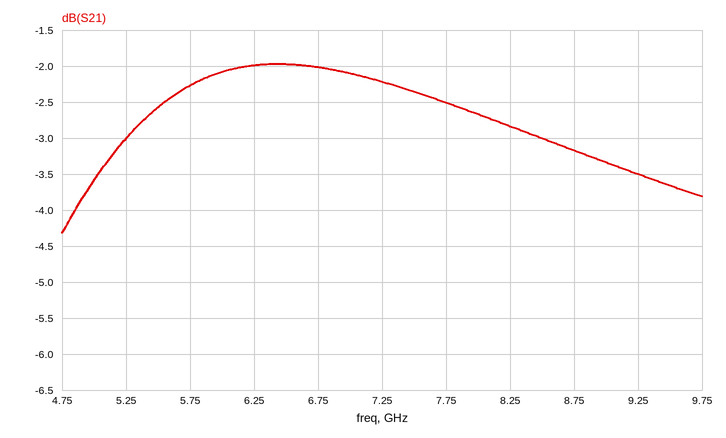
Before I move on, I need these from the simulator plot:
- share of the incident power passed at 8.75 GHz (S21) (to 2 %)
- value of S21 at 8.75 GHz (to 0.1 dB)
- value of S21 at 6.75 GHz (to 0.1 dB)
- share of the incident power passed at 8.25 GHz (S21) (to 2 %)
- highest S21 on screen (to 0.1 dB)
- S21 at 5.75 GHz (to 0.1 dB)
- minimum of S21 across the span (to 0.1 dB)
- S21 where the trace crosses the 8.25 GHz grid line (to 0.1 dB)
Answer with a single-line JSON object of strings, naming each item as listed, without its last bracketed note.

{"share of the incident power passed at 8.75 GHz (S21)": "48 %", "value of S21 at 8.75 GHz": "-3.2 dB", "value of S21 at 6.75 GHz": "-2.0 dB", "share of the incident power passed at 8.25 GHz (S21)": "52 %", "highest S21 on screen": "-2.0 dB", "S21 at 5.75 GHz": "-2.3 dB", "minimum of S21 across the span": "-4.3 dB", "S21 where the trace crosses the 8.25 GHz grid line": "-2.8 dB"}
